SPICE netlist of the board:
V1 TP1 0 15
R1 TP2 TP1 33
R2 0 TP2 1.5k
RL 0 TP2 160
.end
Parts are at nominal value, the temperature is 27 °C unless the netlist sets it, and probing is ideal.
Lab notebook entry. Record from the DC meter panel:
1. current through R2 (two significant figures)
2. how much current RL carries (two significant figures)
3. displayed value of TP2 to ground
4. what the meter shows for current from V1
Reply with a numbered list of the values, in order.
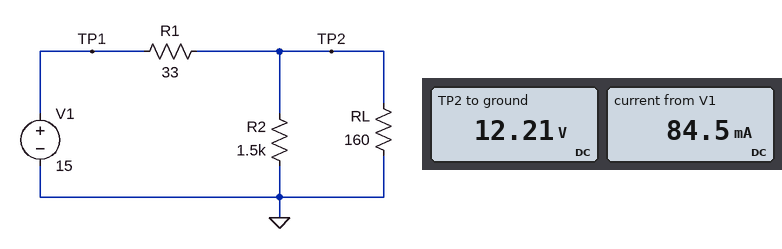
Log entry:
1. 8.1 mA
2. 76 mA
3. 12.21 V
4. 84.5 mA
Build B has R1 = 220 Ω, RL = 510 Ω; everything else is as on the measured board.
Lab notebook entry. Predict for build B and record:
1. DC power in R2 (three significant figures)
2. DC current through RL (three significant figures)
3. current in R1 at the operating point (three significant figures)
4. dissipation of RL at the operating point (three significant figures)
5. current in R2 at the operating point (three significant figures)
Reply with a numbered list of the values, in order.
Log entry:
1. 60.2 mW
2. 18.6 mA
3. 25.0 mA
4. 177 mW
5. 6.34 mA
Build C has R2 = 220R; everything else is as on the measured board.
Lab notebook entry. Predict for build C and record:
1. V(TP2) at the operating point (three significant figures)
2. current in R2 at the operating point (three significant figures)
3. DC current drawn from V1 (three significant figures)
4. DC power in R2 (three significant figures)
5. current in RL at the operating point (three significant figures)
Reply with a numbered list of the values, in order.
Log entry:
1. 11.1 V
2. 50.3 mA
3. 119 mA
4. 556 mW
5. 69.1 mA
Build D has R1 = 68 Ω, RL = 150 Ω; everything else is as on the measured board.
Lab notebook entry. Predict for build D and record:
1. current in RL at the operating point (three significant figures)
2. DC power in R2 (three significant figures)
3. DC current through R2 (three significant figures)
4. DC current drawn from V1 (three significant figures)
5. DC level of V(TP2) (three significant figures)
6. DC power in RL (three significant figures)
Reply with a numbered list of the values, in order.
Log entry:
1. 66.7 mA
2. 66.8 mW
3. 6.67 mA
4. 73.4 mA
5. 10.0 V
6. 668 mW
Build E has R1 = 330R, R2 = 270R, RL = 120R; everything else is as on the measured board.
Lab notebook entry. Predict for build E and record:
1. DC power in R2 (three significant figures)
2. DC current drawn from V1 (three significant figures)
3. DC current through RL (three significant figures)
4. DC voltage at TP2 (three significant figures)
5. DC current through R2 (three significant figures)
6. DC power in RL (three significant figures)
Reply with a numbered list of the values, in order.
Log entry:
1. 33.7 mW
2. 36.3 mA
3. 25.1 mA
4. 3.02 V
5. 11.2 mA
6. 75.8 mW
